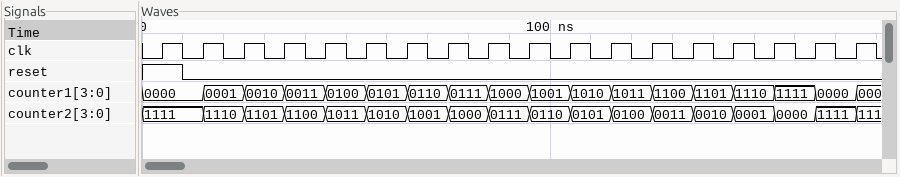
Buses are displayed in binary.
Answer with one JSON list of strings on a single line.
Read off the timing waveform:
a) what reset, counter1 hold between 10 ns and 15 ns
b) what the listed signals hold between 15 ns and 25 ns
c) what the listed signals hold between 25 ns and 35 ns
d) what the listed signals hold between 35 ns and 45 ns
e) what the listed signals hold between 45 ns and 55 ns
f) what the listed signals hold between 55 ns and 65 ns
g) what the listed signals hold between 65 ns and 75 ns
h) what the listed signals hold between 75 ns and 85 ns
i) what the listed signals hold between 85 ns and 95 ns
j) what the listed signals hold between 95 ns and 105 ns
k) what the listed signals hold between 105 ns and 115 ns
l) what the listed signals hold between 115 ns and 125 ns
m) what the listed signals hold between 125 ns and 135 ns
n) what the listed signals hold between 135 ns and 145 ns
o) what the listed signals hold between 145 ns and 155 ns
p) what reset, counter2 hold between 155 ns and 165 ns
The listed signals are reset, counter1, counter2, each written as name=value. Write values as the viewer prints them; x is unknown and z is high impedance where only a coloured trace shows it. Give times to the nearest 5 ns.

["reset=0, counter1=0000", "reset=0, counter1=0001, counter2=1110", "reset=0, counter1=0010, counter2=1101", "reset=0, counter1=0011, counter2=1100", "reset=0, counter1=0100, counter2=1011", "reset=0, counter1=0101, counter2=1010", "reset=0, counter1=0110, counter2=1001", "reset=0, counter1=0111, counter2=1000", "reset=0, counter1=1000, counter2=0111", "reset=0, counter1=1001, counter2=0110", "reset=0, counter1=1010, counter2=0101", "reset=0, counter1=1011, counter2=0100", "reset=0, counter1=1100, counter2=0011", "reset=0, counter1=1101, counter2=0010", "reset=0, counter1=1110, counter2=0001", "reset=0, counter2=0000"]
